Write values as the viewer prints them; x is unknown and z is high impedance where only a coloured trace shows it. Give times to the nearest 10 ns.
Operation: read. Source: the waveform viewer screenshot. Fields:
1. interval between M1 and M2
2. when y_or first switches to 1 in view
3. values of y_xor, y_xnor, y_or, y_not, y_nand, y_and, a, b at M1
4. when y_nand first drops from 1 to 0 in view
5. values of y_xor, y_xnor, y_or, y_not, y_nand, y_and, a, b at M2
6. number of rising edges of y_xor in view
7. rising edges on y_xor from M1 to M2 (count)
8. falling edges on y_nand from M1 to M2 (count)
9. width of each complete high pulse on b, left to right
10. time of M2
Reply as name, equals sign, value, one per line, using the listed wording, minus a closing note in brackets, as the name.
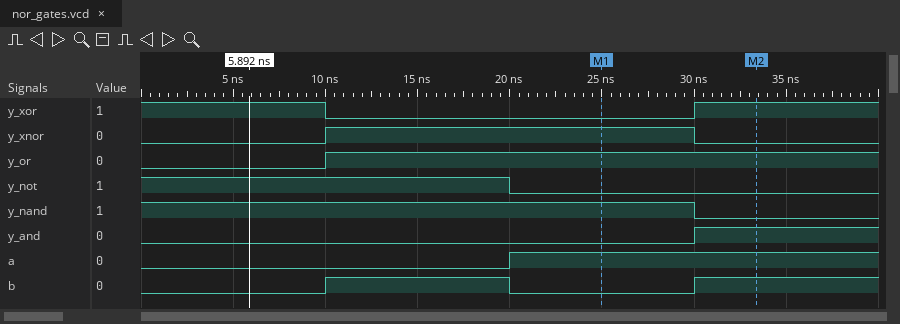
interval between M1 and M2 = 10 ns
when y_or first switches to 1 in view = 10 ns
values of y_xor, y_xnor, y_or, y_not, y_nand, y_and, a, b at M1 = y_xor=0, y_xnor=1, y_or=1, y_not=0, y_nand=1, y_and=0, a=1, b=0
when y_nand first drops from 1 to 0 in view = 30 ns
values of y_xor, y_xnor, y_or, y_not, y_nand, y_and, a, b at M2 = y_xor=1, y_xnor=0, y_or=1, y_not=0, y_nand=0, y_and=1, a=1, b=1
number of rising edges of y_xor in view = 1
rising edges on y_xor from M1 to M2 = 1
falling edges on y_nand from M1 to M2 = 1
width of each complete high pulse on b, left to right = 10 ns
time of M2 = 30 ns
